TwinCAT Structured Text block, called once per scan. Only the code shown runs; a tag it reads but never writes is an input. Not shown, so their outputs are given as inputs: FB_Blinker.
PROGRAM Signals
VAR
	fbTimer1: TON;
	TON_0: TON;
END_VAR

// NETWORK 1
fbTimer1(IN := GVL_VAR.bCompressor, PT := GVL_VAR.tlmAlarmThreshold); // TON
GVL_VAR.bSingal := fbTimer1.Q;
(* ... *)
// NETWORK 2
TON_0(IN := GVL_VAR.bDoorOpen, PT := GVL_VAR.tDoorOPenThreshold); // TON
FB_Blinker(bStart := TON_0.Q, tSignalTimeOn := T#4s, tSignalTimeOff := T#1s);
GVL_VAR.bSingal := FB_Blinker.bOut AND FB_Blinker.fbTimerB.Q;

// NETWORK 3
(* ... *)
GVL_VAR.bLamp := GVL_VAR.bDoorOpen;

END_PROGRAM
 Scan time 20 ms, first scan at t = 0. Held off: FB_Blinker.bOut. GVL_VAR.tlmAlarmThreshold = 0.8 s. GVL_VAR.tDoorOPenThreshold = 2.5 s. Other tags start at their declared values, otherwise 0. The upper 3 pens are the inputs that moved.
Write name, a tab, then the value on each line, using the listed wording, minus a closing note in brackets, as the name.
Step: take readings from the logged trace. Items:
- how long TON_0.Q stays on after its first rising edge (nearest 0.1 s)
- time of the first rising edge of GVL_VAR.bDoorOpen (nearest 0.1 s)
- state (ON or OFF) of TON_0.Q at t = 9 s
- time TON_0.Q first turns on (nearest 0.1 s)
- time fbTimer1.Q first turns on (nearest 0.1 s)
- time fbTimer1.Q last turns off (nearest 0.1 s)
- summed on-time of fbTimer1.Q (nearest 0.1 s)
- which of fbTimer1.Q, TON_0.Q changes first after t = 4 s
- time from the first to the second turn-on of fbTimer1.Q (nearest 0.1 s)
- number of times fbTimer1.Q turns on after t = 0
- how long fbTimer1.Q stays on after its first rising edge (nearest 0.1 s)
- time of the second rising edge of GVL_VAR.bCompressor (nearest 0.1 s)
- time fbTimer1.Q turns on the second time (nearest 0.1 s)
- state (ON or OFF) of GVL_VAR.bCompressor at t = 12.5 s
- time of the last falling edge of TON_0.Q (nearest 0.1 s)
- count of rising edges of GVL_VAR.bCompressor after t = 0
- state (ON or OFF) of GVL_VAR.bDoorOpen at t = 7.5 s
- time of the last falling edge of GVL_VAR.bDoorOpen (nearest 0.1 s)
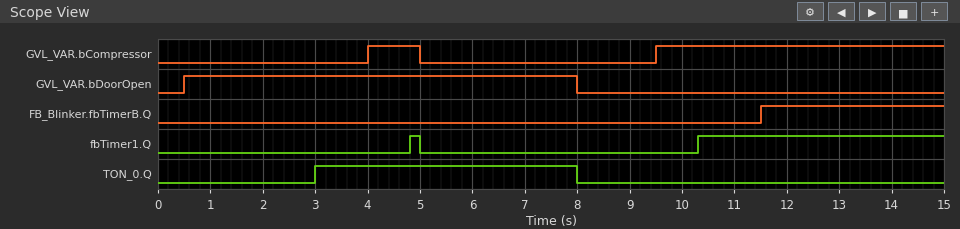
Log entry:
how long TON_0.Q stays on after its first rising edge	5.0 s
time of the first rising edge of GVL_VAR.bDoorOpen	0.5 s
state (ON or OFF) of TON_0.Q at t = 9 s	OFF
time TON_0.Q first turns on	3.0 s
time fbTimer1.Q first turns on	4.8 s
time fbTimer1.Q last turns off	5.0 s
summed on-time of fbTimer1.Q	4.9 s
which of fbTimer1.Q, TON_0.Q changes first after t = 4 s	fbTimer1.Q
time from the first to the second turn-on of fbTimer1.Q	5.5 s
number of times fbTimer1.Q turns on after t = 0	2
how long fbTimer1.Q stays on after its first rising edge	0.2 s
time of the second rising edge of GVL_VAR.bCompressor	9.5 s
time fbTimer1.Q turns on the second time	10.3 s
state (ON or OFF) of GVL_VAR.bCompressor at t = 12.5 s	ON
time of the last falling edge of TON_0.Q	8.0 s
count of rising edges of GVL_VAR.bCompressor after t = 0	2
state (ON or OFF) of GVL_VAR.bDoorOpen at t = 7.5 s	ON
time of the last falling edge of GVL_VAR.bDoorOpen	8.0 s
